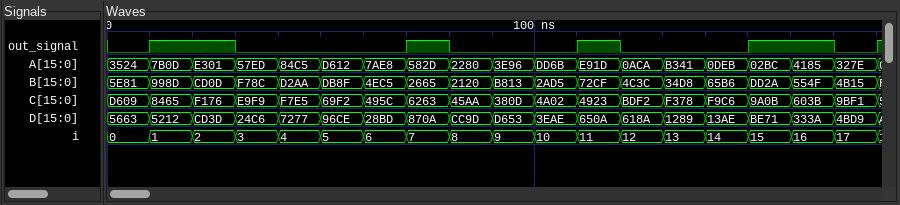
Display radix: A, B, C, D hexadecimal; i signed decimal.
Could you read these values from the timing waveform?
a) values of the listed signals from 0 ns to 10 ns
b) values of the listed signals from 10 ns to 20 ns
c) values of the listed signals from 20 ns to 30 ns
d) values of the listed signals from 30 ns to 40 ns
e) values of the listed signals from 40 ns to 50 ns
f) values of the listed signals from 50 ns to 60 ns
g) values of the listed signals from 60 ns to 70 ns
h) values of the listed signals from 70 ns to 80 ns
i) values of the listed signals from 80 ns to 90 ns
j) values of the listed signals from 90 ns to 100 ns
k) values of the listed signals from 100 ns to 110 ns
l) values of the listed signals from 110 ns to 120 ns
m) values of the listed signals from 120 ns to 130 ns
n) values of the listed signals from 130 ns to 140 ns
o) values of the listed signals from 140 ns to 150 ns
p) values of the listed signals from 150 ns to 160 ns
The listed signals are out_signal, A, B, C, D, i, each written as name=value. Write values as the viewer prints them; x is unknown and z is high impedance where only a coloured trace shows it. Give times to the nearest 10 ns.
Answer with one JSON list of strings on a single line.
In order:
["out_signal=0, A=3524, B=5E81, C=D609, D=5663, i=0", "out_signal=1, A=7B0D, B=998D, C=8465, D=5212, i=1", "out_signal=1, A=E301, B=CD0D, C=F176, D=CD3D, i=2", "out_signal=0, A=57ED, B=F78C, C=E9F9, D=24C6, i=3", "out_signal=0, A=84C5, B=D2AA, C=F7E5, D=7277, i=4", "out_signal=0, A=D612, B=DB8F, C=69F2, D=96CE, i=5", "out_signal=0, A=7AE8, B=4EC5, C=495C, D=28BD, i=6", "out_signal=1, A=582D, B=2665, C=6263, D=870A, i=7", "out_signal=0, A=2280, B=2120, C=45AA, D=CC9D, i=8", "out_signal=0, A=3E96, B=B813, C=380D, D=D653, i=9", "out_signal=0, A=DD6B, B=2AD5, C=4A02, D=3EAE, i=10", "out_signal=1, A=E91D, B=72CF, C=4923, D=650A, i=11", "out_signal=0, A=0ACA, B=4C3C, C=BDF2, D=618A, i=12", "out_signal=0, A=B341, B=34D8, C=F378, D=1289, i=13", "out_signal=0, A=0DEB, B=65B6, C=F9C6, D=13AE, i=14", "out_signal=1, A=02BC, B=DD2A, C=9A0B, D=BE71, i=15"]
